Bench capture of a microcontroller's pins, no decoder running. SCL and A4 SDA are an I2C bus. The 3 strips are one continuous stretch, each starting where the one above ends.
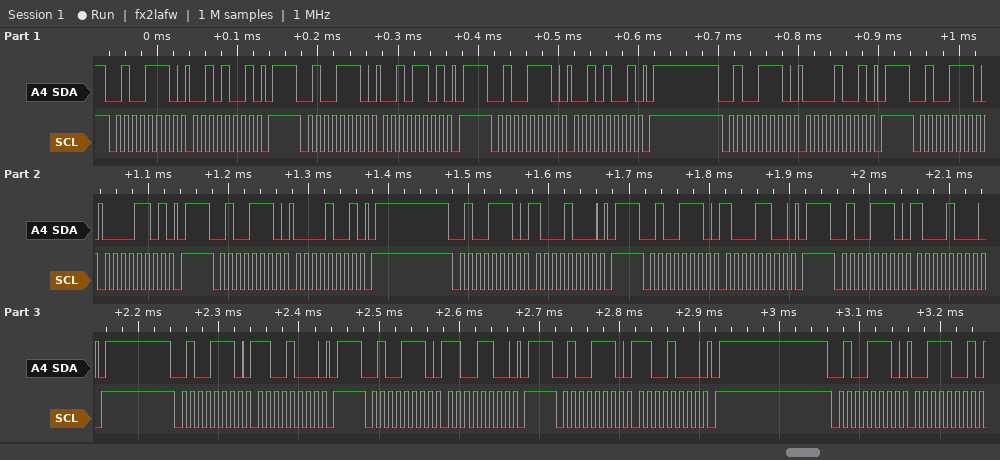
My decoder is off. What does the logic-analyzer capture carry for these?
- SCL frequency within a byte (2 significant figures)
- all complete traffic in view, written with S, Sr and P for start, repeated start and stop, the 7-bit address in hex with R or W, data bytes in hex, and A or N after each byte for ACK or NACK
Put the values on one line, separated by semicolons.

100 kHz; S 27W A 29 A P S 27W A 2D A P S 27W A 29 A P S 27W A 09 A P S 27W A 0D A P S 27W A 09 A P S 27W A 88 A P S 27W A 8C A P S 27W A 88 A P S 27W A C8 A P S 27W A CC A P S 27W A C8 A P S 27W A 39 A
